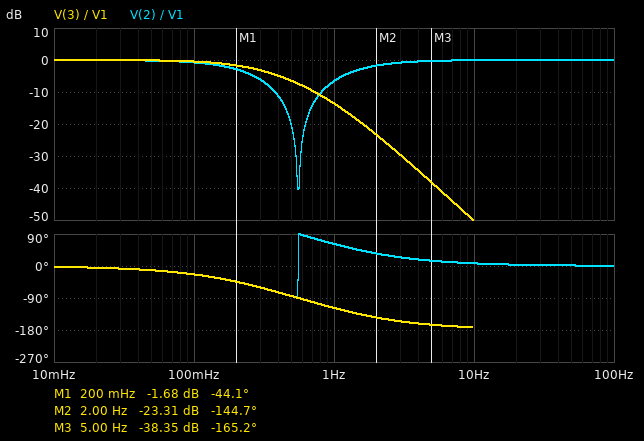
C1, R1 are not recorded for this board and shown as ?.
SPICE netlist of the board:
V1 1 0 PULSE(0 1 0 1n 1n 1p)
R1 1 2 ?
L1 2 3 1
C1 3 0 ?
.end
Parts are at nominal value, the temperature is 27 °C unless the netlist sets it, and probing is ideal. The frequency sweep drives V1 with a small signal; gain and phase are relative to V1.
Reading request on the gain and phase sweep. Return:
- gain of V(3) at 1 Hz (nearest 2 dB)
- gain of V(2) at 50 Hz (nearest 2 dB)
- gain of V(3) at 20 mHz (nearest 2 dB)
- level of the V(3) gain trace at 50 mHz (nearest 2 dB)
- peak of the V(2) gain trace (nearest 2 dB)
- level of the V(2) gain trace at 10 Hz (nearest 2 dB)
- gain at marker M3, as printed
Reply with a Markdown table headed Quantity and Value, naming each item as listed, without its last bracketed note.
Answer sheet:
| Quantity | Value |
|---|---|
| gain of V(3) at 1 Hz | -14 dB |
| gain of V(2) at 50 Hz | 0 dB |
| gain of V(3) at 20 mHz | 0 dB |
| level of the V(3) gain trace at 50 mHz | 0 dB |
| peak of the V(2) gain trace | 0 dB |
| level of the V(2) gain trace at 10 Hz | 0 dB |
| gain at marker M3, as printed | -38.35 dB |
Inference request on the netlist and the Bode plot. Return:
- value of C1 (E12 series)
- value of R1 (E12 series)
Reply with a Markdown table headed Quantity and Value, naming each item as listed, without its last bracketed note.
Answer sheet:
| Quantity | Value |
|---|---|
| value of C1 | 82 mF |
| value of R1 | 8.2 Ω |
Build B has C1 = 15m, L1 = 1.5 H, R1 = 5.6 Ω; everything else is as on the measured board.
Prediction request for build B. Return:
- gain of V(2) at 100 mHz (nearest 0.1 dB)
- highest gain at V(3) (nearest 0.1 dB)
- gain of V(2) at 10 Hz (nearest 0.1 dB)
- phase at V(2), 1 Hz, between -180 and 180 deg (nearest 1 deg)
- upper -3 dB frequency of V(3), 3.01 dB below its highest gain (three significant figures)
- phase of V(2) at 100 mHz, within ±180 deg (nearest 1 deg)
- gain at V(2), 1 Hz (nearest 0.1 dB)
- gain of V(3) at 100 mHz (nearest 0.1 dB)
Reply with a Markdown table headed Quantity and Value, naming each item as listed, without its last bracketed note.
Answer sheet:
| Quantity | Value |
|---|---|
| gain of V(2) at 100 mHz | 0 dB |
| highest gain at V(3) | 5.4 dB |
| gain of V(2) at 10 Hz | 0 dB |
| phase at V(2), 1 Hz, between -180 and 180 deg | -78 deg |
| upper -3 dB frequency of V(3), 3.01 dB below its highest gain | 1.25 Hz |
| phase of V(2) at 100 mHz, within ±180 deg | -3 deg |
| gain at V(2), 1 Hz | -13.7 dB |
| gain of V(3) at 100 mHz | 0.1 dB |
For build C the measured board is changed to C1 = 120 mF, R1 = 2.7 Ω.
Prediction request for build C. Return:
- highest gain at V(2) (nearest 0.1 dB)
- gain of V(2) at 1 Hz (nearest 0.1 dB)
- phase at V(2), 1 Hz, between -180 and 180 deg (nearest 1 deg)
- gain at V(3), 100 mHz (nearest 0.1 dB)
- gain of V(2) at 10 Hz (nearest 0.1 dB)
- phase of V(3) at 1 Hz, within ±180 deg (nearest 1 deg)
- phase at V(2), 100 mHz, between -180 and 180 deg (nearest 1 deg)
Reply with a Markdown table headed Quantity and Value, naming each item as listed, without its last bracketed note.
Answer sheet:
| Quantity | Value |
|---|---|
| highest gain at V(2) | 0 dB |
| gain of V(2) at 1 Hz | -1.1 dB |
| phase at V(2), 1 Hz, between -180 and 180 deg | 29 deg |
| gain at V(3), 100 mHz | 0.2 dB |
| gain of V(2) at 10 Hz | 0 dB |
| phase of V(3) at 1 Hz, within ±180 deg | -151 deg |
| phase at V(2), 100 mHz, between -180 and 180 deg | -12 deg |
